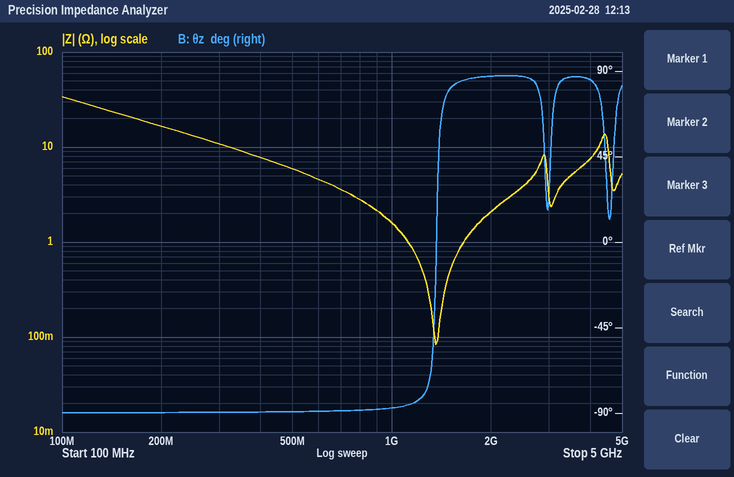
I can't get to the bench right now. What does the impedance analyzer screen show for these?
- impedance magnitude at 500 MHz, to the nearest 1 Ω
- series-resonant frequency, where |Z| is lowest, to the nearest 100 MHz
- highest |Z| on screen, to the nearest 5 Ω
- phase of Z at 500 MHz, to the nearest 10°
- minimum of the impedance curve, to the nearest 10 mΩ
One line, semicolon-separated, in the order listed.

6 Ω; 1.4 GHz; 35 Ω; -90°; 80 mΩ
